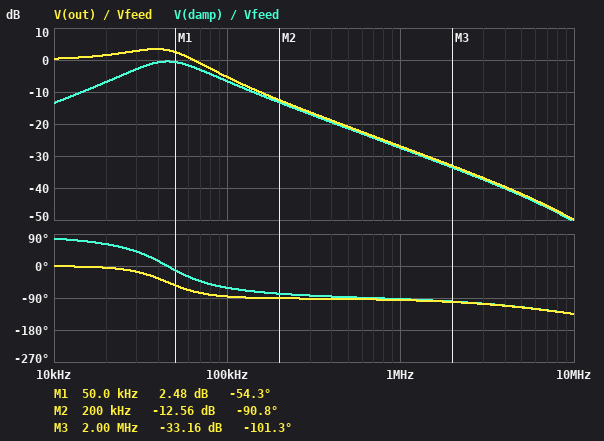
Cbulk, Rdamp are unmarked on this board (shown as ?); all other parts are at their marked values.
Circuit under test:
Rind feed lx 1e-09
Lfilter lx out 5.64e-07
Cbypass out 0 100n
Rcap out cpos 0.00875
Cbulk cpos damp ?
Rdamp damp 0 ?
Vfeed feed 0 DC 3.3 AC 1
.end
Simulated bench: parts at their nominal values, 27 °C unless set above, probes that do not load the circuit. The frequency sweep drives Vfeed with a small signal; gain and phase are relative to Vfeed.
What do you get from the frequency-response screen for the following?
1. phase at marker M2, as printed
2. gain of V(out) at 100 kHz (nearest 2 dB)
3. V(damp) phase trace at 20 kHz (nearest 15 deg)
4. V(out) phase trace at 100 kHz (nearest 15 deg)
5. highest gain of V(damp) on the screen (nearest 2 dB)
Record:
-90.8 deg
-6 dB
60 deg
-90 deg
0 dB
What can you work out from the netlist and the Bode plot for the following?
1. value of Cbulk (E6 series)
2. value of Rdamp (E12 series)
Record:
22 µF
0.15 Ω
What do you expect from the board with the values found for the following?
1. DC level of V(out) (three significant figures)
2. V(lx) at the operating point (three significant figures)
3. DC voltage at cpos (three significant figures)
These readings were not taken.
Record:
3.30 V
3.30 V
3.30 V
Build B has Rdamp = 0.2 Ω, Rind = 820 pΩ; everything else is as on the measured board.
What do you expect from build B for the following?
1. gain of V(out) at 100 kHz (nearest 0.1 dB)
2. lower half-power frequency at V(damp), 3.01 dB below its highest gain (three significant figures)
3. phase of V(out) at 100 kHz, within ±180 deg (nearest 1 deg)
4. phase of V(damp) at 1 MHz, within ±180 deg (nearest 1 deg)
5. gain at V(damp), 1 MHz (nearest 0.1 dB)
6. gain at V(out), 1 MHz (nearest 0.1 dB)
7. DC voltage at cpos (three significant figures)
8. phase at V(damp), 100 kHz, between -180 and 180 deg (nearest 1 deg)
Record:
-4.0 dB
24.6 kHz
-73 deg
-94 deg
-25.0 dB
-24.6 dB
3.30 V
-54 deg
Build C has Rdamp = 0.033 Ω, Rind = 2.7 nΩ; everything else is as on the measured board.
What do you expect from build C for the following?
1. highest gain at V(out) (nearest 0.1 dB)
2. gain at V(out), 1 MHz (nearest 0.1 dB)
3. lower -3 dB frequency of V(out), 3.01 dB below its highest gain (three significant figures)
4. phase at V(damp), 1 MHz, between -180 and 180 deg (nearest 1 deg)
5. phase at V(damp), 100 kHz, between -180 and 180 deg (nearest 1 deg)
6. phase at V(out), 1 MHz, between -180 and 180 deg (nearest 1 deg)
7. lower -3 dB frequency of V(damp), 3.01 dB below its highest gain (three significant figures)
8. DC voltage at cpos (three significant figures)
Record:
12.1 dB
-38.5 dB
38.1 kHz
-91 deg
-82 deg
-101 deg
39.6 kHz
3.30 V
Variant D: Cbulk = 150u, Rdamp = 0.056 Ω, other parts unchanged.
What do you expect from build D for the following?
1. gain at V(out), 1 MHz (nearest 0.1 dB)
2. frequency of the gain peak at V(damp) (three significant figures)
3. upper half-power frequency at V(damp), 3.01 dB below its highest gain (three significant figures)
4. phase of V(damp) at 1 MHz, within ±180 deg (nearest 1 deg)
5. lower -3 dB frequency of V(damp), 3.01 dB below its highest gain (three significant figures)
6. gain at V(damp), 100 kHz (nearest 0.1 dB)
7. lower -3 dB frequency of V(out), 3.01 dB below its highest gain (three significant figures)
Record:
-34.8 dB
17.3 kHz
28.7 kHz
-91 deg
10.4 kHz
-15.9 dB
1.90 kHz
